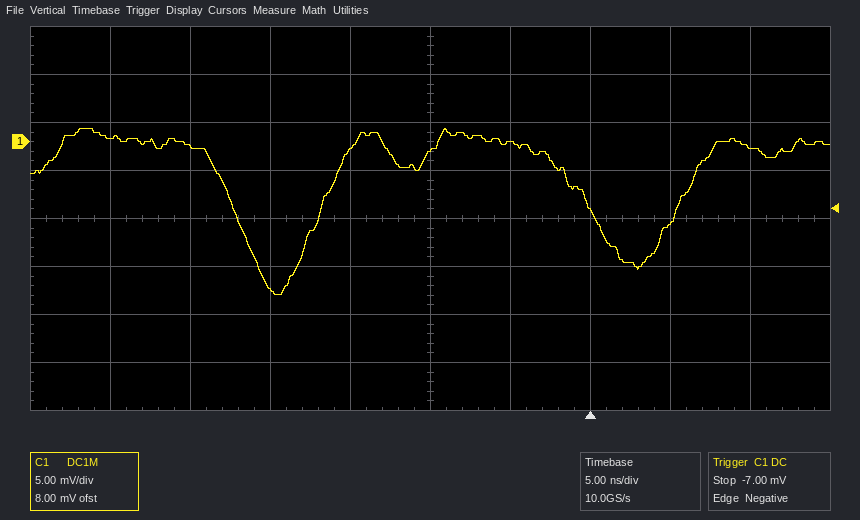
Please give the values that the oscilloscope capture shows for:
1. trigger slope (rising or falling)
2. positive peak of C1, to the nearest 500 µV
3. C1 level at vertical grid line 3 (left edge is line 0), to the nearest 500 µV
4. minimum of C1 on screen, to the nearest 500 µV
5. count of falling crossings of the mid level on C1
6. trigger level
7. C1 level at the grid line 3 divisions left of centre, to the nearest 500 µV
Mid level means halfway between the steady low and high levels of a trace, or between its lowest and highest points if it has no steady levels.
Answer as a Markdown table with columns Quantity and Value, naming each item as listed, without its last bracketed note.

| Quantity | Value |
|---|---|
| trigger slope | falling |
| positive peak of C1, to the nearest 500 µV | 1.5 mV |
| C1 level at vertical grid line 3 (left edge is line 0), to the nearest 500 µV | -15.5 mV |
| minimum of C1 on screen, to the nearest 500 µV | -16.0 mV |
| count of falling crossings of the mid level on C1 | 2 |
| trigger level | -7.00 mV |
| C1 level at the grid line 3 divisions left of centre, to the nearest 500 µV | -500 µV |
